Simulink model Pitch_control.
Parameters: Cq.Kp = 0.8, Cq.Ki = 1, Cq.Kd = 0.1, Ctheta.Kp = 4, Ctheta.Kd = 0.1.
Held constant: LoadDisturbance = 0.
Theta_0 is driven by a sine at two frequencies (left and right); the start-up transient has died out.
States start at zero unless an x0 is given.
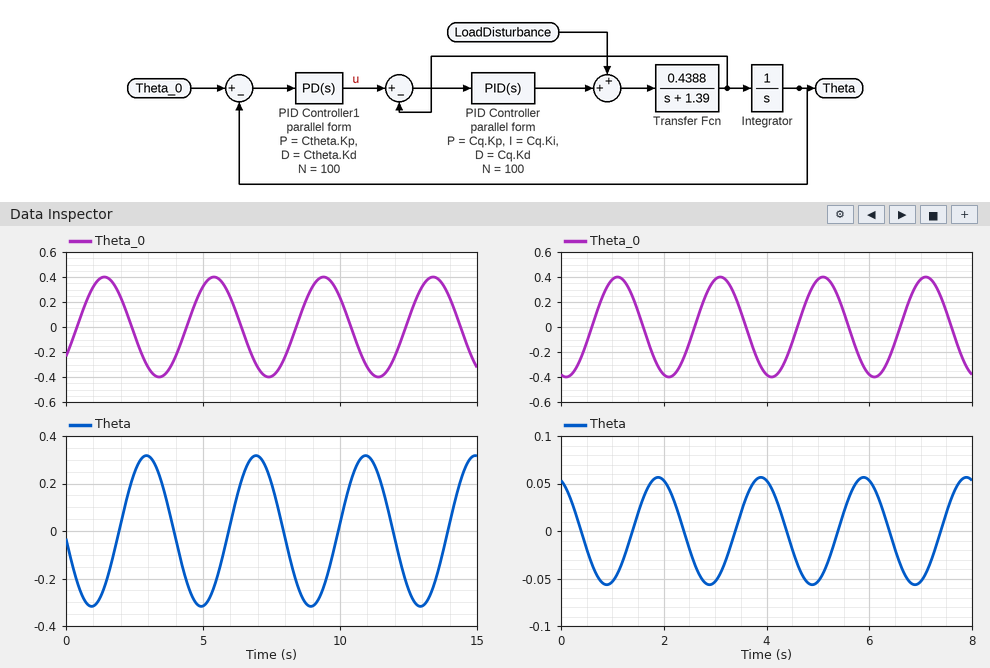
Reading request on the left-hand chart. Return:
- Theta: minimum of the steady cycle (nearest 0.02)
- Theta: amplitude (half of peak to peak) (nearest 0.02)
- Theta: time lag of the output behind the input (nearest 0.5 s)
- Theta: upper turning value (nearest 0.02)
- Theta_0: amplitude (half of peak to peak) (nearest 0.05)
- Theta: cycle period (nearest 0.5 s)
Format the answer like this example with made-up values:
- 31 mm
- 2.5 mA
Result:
- -0.32
- 0.32
- 1.5 s
- 0.32
- 0.40
- 4.0 s
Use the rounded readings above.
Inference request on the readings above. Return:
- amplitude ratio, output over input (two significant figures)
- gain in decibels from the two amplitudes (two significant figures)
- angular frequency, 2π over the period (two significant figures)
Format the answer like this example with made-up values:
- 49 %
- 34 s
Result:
- 0.80
- -1.9 dB
- 1.6 rad/s
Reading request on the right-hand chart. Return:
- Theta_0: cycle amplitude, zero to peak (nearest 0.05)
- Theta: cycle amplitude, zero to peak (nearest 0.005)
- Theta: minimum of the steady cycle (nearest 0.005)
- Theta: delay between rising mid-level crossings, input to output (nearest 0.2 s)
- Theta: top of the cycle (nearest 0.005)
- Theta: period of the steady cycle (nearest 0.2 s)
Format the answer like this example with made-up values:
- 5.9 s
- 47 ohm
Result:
- 0.40
- 0.055
- -0.055
- 0.8 s
- 0.055
- 2.0 s
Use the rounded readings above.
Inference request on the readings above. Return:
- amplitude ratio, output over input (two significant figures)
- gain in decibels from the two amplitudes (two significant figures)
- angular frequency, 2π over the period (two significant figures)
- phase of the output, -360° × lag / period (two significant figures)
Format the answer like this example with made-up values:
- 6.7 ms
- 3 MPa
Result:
- 0.14
- -17 dB
- 3.1 rad/s
- -140°
